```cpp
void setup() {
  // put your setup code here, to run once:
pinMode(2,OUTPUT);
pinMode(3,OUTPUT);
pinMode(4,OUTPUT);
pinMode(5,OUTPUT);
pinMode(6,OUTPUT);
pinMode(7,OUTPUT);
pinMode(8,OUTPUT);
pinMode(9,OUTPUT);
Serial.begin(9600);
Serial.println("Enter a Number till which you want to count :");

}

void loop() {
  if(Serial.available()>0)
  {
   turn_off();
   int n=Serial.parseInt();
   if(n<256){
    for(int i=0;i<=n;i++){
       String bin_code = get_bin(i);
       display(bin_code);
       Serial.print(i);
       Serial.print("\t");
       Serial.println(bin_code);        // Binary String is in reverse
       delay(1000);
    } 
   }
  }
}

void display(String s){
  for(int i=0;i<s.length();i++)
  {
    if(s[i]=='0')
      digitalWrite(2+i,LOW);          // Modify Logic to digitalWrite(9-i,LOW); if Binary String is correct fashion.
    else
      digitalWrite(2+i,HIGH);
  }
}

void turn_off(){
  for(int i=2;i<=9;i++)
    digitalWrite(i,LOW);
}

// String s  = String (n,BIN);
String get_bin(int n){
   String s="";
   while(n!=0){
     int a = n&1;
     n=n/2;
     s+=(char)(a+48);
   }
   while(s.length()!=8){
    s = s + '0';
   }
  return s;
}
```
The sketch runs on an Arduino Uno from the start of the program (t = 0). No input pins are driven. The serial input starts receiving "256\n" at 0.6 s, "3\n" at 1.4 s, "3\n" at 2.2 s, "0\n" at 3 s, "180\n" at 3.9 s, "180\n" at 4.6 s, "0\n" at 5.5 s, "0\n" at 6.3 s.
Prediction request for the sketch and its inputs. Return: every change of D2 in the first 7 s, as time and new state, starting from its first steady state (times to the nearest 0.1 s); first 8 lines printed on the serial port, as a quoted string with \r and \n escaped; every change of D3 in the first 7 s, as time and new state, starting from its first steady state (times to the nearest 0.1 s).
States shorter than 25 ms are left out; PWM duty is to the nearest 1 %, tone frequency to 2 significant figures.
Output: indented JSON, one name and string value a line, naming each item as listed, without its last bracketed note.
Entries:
{
  "every change of D2 in the first 7 s, as time and new state, starting from its first steady state": "0 s low; 2.4 s high; 3.4 s low; 4.4 s high; 5.4 s low; 6.4 s high",
  "first 8 lines printed on the serial port, as a quoted string with \\r and \\n escaped": "\"Enter a Number till which you want to count :\\r\\n0\\t00000000\\r\\n1\\t10000000\\r\\n2\\t01000000\\r\\n3\\t11000000\\r\\n0\\t00000000\\r\\n1\\t10000000\\r\\n2\\t01000000\\r\\n\"",
  "every change of D3 in the first 7 s, as time and new state, starting from its first steady state": "0 s low; 3.4 s high; 5.4 s low"
}
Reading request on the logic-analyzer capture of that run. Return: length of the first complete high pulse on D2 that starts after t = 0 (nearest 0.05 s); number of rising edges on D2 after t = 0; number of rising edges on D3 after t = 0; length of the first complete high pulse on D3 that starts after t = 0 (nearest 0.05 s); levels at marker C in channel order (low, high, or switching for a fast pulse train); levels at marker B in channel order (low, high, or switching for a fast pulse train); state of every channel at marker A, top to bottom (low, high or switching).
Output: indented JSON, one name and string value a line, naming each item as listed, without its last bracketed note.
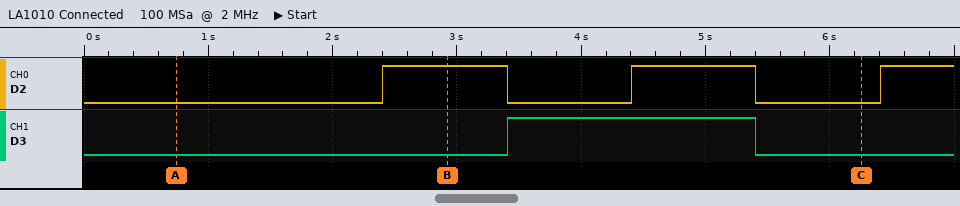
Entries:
{
  "length of the first complete high pulse on D2 that starts after t = 0": "1.00 s",
  "number of rising edges on D2 after t = 0": "3",
  "number of rising edges on D3 after t = 0": "1",
  "length of the first complete high pulse on D3 that starts after t = 0": "2.00 s",
  "levels at marker C in channel order": "D2 low, D3 low",
  "levels at marker B in channel order": "D2 high, D3 low",
  "state of every channel at marker A, top to bottom": "D2 low, D3 low"
}
